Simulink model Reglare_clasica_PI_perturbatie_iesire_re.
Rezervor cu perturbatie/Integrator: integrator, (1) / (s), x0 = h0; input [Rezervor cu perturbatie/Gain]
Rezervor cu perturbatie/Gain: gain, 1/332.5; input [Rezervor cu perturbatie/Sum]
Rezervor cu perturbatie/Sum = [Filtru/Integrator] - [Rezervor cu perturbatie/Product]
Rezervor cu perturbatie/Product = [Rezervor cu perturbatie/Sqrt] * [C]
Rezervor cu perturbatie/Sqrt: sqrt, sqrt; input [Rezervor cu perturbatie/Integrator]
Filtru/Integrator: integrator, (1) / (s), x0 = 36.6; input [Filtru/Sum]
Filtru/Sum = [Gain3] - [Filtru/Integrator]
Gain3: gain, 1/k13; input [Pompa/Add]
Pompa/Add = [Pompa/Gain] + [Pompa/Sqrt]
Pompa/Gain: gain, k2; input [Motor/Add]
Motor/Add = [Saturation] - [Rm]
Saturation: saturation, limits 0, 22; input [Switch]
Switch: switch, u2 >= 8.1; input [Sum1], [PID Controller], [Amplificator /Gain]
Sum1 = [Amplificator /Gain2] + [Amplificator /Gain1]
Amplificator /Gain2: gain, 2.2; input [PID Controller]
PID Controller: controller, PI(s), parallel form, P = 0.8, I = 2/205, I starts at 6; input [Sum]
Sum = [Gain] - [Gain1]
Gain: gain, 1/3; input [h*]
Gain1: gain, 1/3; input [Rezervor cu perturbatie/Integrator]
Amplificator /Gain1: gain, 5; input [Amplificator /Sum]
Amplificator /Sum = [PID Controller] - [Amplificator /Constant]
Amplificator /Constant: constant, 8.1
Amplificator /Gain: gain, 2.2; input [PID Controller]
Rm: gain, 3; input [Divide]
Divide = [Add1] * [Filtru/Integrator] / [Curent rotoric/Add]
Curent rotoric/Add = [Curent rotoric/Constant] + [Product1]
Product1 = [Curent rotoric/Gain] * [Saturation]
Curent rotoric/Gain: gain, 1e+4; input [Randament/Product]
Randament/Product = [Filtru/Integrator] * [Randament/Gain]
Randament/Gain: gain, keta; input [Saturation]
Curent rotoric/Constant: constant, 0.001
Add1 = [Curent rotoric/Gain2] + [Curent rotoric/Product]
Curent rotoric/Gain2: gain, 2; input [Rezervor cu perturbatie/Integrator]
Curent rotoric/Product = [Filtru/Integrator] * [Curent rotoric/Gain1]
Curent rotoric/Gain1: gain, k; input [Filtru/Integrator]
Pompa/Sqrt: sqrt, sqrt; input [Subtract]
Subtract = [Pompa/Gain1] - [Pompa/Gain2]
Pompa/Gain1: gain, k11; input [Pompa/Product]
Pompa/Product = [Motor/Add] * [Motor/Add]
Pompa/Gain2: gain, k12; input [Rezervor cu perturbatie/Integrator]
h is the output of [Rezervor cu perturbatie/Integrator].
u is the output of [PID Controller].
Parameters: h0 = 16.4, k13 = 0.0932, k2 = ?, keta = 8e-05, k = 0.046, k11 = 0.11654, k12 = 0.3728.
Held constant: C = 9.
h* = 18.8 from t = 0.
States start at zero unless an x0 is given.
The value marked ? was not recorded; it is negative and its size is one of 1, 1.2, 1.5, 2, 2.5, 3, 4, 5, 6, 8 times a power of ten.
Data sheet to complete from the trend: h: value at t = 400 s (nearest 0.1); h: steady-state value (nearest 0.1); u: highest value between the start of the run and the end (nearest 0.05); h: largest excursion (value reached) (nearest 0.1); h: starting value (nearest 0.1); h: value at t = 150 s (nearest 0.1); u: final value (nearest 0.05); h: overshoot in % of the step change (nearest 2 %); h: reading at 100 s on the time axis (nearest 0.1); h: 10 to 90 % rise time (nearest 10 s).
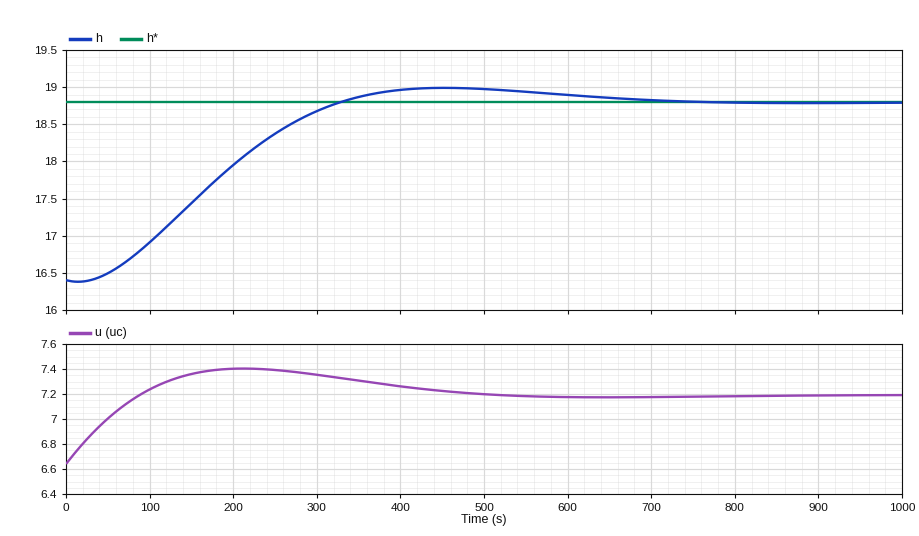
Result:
19.0
18.8
7.40
19.0
16.4
17.4
7.20
8 %
16.9
210 s
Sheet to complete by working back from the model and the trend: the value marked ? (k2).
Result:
-0.03
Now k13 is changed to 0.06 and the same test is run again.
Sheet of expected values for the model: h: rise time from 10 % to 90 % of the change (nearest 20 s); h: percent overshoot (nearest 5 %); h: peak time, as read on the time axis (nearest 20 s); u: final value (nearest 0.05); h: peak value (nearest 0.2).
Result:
80 s
20 %
200 s
6.05
19.2
